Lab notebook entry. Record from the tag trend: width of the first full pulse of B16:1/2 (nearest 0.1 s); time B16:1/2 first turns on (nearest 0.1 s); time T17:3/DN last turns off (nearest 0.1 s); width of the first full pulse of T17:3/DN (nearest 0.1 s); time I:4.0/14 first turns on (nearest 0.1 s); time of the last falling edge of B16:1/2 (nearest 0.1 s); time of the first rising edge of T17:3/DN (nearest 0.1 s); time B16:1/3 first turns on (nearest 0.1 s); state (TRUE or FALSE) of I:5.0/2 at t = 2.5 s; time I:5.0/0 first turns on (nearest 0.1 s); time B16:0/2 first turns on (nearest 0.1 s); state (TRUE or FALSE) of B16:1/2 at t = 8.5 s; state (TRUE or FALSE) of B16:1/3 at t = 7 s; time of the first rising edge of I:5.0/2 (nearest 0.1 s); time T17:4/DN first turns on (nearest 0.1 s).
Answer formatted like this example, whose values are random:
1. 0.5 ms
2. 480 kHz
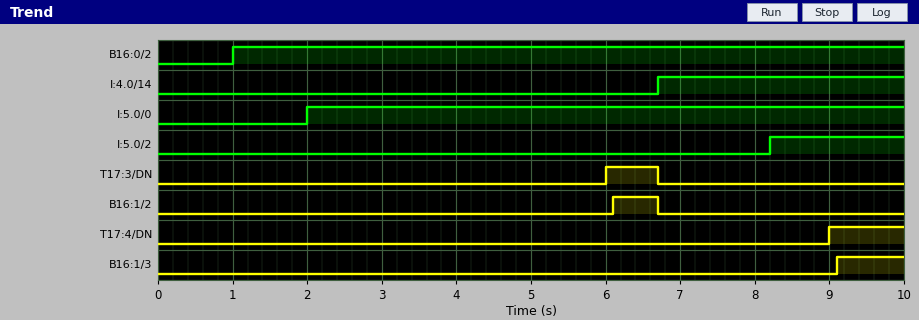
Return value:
1. 0.6 s
2. 6.1 s
3. 6.7 s
4. 0.7 s
5. 6.7 s
6. 6.7 s
7. 6.0 s
8. 9.1 s
9. FALSE
10. 2.0 s
11. 1.0 s
12. FALSE
13. FALSE
14. 8.2 s
15. 9.0 s
